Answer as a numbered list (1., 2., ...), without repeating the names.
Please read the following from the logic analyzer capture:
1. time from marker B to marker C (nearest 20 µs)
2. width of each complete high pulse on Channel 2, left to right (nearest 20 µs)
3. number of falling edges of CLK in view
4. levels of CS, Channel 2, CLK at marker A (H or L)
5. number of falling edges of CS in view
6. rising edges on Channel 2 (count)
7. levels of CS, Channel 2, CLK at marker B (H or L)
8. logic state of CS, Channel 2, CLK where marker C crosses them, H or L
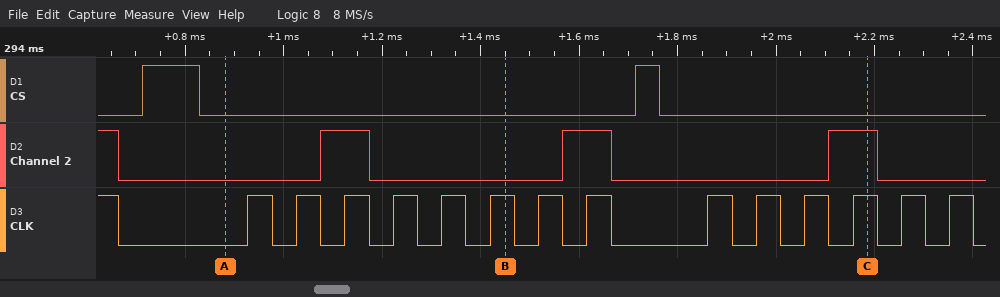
1. 740 µs
2. 100 µs, 100 µs, 100 µs
3. 15
4. CS=L, Channel 2=L, CLK=L
5. 2
6. 3
7. CS=L, Channel 2=L, CLK=H
8. CS=L, Channel 2=H, CLK=H
